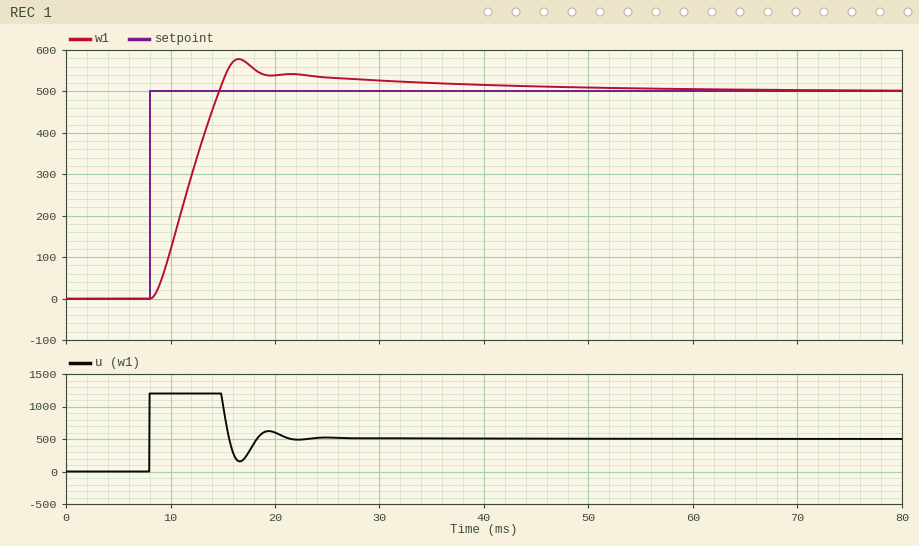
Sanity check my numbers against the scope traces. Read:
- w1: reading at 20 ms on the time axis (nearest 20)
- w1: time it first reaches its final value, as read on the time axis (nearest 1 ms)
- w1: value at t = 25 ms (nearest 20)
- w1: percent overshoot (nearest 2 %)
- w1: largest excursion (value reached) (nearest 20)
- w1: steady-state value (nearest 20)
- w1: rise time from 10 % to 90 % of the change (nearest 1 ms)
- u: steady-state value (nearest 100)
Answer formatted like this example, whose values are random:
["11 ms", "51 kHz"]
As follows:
["540", "15 ms", "540", "16 %", "580", "500", "5 ms", "500"]
